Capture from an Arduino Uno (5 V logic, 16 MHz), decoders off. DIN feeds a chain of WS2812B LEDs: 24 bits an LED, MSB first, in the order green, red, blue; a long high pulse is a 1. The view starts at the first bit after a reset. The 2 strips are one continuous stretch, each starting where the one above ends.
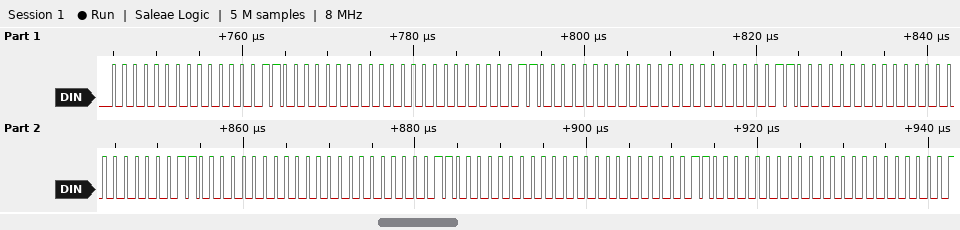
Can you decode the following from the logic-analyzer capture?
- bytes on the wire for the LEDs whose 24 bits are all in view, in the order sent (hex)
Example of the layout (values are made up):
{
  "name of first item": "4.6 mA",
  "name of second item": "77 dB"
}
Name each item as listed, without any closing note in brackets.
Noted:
{
  "bytes on the wire for the LEDs whose 24 bits are all in view, in the order sent": "00 03 00 00 03 00 00 03 00 00 03 00 00 03 00 00 03 00"
}
